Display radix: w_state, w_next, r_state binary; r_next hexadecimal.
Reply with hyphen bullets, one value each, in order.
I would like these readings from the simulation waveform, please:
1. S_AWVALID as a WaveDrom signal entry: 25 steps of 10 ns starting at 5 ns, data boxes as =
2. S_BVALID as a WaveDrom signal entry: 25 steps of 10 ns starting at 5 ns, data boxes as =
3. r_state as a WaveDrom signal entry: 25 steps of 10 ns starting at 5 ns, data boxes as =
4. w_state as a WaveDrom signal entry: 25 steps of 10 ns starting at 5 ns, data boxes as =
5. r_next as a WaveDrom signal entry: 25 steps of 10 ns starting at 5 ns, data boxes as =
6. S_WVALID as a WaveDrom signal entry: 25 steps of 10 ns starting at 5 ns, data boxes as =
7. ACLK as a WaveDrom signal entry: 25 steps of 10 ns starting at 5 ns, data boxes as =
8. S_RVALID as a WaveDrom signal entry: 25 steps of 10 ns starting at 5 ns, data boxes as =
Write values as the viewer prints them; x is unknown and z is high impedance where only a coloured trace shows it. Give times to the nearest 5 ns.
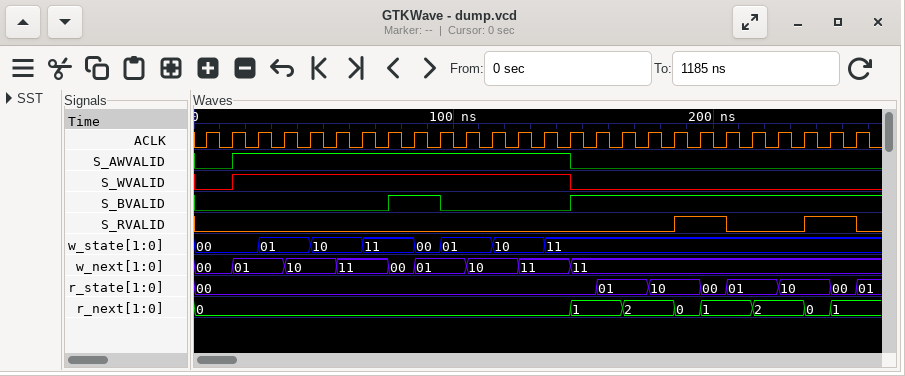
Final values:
- {name: 'S_AWVALID', wave: '01............0..........'}
- {name: 'S_BVALID', wave: '0......1.0....1..........'}
- {name: 'r_state', wave: '=..............=.=.==.=.=', data: '00 01 10 00 01 10 00'}
- {name: 'w_state', wave: '=.=.=.=.==.=.=...........', data: '00 01 10 11 00 01 10 11'}
- {name: 'r_next', wave: '=.............=.=.==.=.==', data: '0 1 2 0 1 2 0 1'}
- {name: 'S_WVALID', wave: '01............0..........'}
- {name: 'ACLK', wave: 'p........................'}
- {name: 'S_RVALID', wave: '0.................1.0..1.'}
